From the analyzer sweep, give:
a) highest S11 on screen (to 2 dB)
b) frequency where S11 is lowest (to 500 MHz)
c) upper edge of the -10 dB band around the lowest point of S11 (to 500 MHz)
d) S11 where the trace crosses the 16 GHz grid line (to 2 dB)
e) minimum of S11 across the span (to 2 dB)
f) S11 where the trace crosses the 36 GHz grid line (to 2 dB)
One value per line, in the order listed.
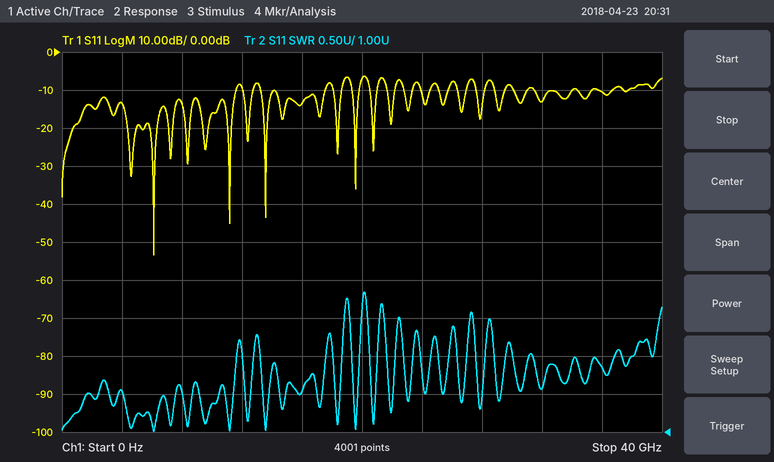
-6 dB
6.0 GHz
11.5 GHz
-14 dB
-54 dB
-10 dB
